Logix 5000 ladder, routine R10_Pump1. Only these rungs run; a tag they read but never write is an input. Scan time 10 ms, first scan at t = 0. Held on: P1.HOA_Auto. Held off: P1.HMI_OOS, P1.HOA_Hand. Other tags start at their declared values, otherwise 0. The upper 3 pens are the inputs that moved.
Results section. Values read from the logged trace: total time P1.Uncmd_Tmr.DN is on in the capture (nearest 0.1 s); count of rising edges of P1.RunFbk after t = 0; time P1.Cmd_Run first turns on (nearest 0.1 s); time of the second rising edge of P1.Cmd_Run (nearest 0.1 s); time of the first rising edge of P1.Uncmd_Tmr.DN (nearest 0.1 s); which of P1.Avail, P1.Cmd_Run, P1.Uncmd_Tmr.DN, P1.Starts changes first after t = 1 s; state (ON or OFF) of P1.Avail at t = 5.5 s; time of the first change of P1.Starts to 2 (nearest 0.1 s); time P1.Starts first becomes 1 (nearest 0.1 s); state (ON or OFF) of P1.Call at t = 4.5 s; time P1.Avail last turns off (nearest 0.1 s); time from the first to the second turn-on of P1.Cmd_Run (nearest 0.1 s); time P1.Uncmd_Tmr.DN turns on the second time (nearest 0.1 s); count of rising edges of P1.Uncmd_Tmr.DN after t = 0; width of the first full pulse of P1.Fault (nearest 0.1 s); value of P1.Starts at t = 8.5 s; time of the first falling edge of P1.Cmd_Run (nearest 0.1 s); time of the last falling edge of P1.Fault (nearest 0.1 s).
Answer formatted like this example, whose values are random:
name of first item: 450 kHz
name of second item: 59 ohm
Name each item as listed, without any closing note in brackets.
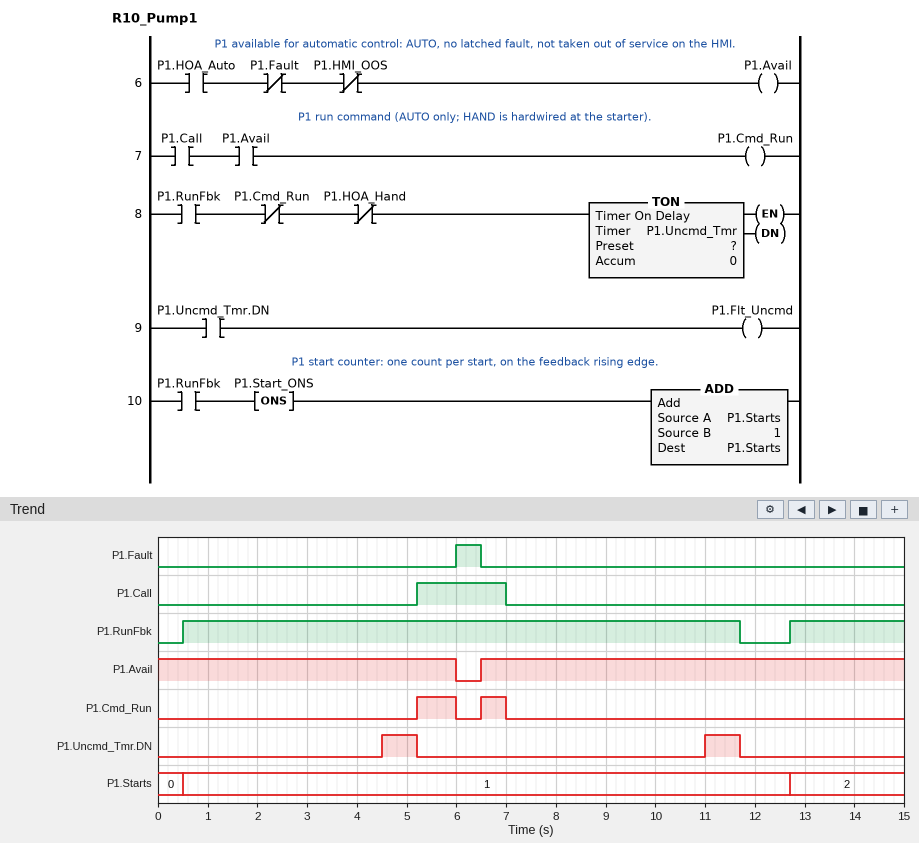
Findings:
total time P1.Uncmd_Tmr.DN is on in the capture: 1.4 s
count of rising edges of P1.RunFbk after t = 0: 2
time P1.Cmd_Run first turns on: 5.2 s
time of the second rising edge of P1.Cmd_Run: 6.5 s
time of the first rising edge of P1.Uncmd_Tmr.DN: 4.5 s
which of P1.Avail, P1.Cmd_Run, P1.Uncmd_Tmr.DN, P1.Starts changes first after t = 1 s: P1.Uncmd_Tmr.DN
state (ON or OFF) of P1.Avail at t = 5.5 s: ON
time of the first change of P1.Starts to 2: 12.7 s
time P1.Starts first becomes 1: 0.5 s
state (ON or OFF) of P1.Call at t = 4.5 s: OFF
time P1.Avail last turns off: 6.0 s
time from the first to the second turn-on of P1.Cmd_Run: 1.3 s
time P1.Uncmd_Tmr.DN turns on the second time: 11.0 s
count of rising edges of P1.Uncmd_Tmr.DN after t = 0: 2
width of the first full pulse of P1.Fault: 0.5 s
value of P1.Starts at t = 8.5 s: 1
time of the first falling edge of P1.Cmd_Run: 6.0 s
time of the last falling edge of P1.Fault: 6.5 s
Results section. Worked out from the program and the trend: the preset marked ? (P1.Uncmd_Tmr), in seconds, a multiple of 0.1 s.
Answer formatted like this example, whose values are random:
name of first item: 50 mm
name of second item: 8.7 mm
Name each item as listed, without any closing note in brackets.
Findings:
the preset marked ? (P1.Uncmd_Tmr), in seconds, a multiple of 0.1 s: 4.0 s
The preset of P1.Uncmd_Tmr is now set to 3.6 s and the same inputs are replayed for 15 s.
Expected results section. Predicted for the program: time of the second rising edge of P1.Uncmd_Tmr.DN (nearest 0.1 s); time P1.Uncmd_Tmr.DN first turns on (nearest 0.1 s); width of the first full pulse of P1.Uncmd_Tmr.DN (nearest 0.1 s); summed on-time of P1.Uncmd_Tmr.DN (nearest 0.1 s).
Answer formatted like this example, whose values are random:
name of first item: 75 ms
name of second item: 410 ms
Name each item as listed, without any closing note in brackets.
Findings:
time of the second rising edge of P1.Uncmd_Tmr.DN: 10.6 s
time P1.Uncmd_Tmr.DN first turns on: 4.1 s
width of the first full pulse of P1.Uncmd_Tmr.DN: 1.1 s
summed on-time of P1.Uncmd_Tmr.DN: 2.2 s
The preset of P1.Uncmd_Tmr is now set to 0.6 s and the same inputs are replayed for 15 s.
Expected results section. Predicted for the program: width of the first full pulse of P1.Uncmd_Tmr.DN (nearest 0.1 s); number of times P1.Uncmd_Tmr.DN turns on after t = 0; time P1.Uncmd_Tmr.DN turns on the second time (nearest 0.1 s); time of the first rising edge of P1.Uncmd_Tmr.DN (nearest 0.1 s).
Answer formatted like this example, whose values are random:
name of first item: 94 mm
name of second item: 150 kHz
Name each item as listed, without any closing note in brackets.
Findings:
width of the first full pulse of P1.Uncmd_Tmr.DN: 4.1 s
number of times P1.Uncmd_Tmr.DN turns on after t = 0: 3
time P1.Uncmd_Tmr.DN turns on the second time: 7.6 s
time of the first rising edge of P1.Uncmd_Tmr.DN: 1.1 s
